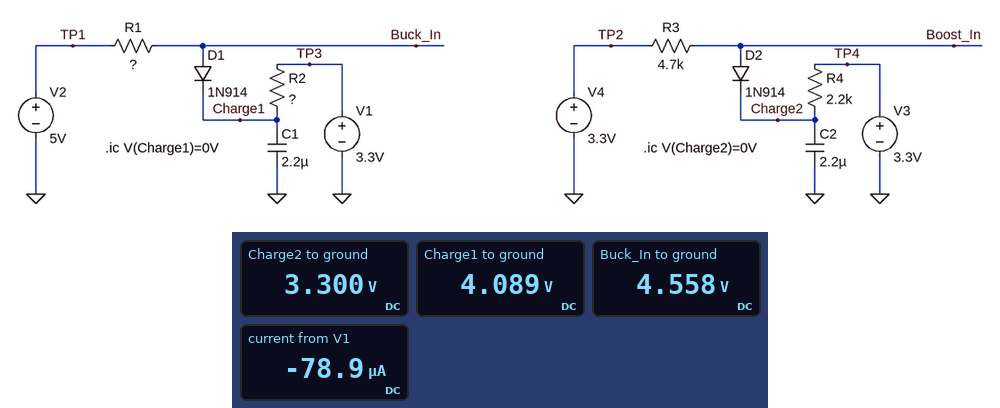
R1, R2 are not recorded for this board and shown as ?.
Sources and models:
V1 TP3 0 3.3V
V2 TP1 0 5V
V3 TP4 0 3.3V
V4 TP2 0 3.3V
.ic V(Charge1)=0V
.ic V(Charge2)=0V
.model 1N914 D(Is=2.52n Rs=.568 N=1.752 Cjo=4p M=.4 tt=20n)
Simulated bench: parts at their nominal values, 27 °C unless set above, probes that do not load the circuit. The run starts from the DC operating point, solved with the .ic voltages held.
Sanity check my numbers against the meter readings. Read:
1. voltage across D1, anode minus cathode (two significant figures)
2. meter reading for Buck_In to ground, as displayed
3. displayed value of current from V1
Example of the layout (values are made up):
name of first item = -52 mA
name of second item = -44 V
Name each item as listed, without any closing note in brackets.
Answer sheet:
voltage across D1, anode minus cathode = 470 mV
meter reading for Buck_In to ground, as displayed = 4.558 V
displayed value of current from V1 = -78.9 µA
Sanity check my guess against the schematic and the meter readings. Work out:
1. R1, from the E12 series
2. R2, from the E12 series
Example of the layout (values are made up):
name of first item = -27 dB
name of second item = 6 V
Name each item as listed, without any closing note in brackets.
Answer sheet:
R1, from the E12 series = 5.6 kΩ
R2, from the E12 series = 10 kΩ
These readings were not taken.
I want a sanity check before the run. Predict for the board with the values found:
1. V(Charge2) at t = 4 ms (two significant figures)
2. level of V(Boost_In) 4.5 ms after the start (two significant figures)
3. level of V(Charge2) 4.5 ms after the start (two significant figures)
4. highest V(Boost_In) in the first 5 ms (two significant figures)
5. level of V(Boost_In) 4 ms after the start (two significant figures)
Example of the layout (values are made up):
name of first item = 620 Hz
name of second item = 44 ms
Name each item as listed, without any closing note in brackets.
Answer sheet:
V(Charge2) at t = 4 ms = 2.2 V
level of V(Boost_In) 4.5 ms after the start = 2.8 V
level of V(Charge2) 4.5 ms after the start = 2.3 V
highest V(Boost_In) in the first 5 ms = 2.9 V
level of V(Boost_In) 4 ms after the start = 2.7 V
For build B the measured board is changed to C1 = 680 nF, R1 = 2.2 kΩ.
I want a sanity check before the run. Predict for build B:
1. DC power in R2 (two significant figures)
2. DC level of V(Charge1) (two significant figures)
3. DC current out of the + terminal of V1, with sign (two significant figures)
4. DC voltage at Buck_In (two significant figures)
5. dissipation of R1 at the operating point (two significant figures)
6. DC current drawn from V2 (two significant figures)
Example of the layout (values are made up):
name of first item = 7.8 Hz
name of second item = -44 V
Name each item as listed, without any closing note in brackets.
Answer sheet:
DC power in R2 = 100 µW
DC level of V(Charge1) = 4.3 V
DC current out of the + terminal of V1, with sign = -100 µA
DC voltage at Buck_In = 4.8 V
dissipation of R1 at the operating point = 22 µW
DC current drawn from V2 = 100 µA
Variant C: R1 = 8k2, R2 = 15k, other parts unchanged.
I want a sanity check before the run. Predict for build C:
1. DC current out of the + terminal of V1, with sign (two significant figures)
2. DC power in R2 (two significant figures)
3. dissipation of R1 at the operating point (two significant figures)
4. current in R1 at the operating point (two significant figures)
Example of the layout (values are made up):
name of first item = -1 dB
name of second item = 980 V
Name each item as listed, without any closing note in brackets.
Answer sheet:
DC current out of the + terminal of V1, with sign = -54 µA
DC power in R2 = 43 µW
dissipation of R1 at the operating point = 24 µW
current in R1 at the operating point = 54 µA
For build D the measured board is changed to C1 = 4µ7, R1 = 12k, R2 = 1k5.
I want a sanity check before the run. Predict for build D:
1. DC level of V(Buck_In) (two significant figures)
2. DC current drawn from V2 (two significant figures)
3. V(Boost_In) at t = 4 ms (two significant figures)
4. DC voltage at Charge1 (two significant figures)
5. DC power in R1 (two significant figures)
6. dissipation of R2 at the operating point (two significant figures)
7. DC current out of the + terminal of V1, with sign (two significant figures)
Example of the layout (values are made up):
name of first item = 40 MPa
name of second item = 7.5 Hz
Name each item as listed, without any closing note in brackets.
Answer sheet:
DC level of V(Buck_In) = 3.9 V
DC current drawn from V2 = 91 µA
V(Boost_In) at t = 4 ms = 2.7 V
DC voltage at Charge1 = 3.4 V
DC power in R1 = 99 µW
dissipation of R2 at the operating point = 12 µW
DC current out of the + terminal of V1, with sign = -91 µA
